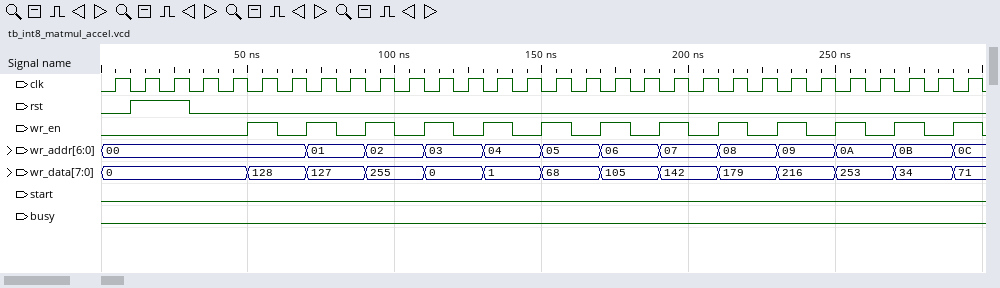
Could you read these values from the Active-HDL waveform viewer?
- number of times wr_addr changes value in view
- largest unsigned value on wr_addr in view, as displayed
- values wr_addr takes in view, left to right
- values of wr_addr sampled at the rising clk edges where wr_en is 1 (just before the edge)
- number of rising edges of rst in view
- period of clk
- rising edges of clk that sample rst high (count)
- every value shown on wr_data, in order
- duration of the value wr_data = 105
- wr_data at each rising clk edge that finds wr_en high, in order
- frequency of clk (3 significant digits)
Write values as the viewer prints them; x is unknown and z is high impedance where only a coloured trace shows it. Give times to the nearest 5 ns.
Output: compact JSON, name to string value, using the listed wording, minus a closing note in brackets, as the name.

{"number of times wr_addr changes value in view": "12", "largest unsigned value on wr_addr in view, as displayed": "0C", "values wr_addr takes in view, left to right": "00, 01, 02, 03, 04, 05, 06, 07, 08, 09, 0A, 0B, 0C", "values of wr_addr sampled at the rising clk edges where wr_en is 1": "00, 01, 02, 03, 04, 05, 06, 07, 08, 09, 0A, 0B, 0C", "number of rising edges of rst in view": "1", "period of clk": "10 ns", "rising edges of clk that sample rst high": "2", "every value shown on wr_data, in order": "0, 128, 127, 255, 0, 1, 68, 105, 142, 179, 216, 253, 34, 71", "duration of the value wr_data = 105": "20 ns", "wr_data at each rising clk edge that finds wr_en high, in order": "128, 127, 255, 0, 1, 68, 105, 142, 179, 216, 253, 34, 71", "frequency of clk": "100 MHz"}
